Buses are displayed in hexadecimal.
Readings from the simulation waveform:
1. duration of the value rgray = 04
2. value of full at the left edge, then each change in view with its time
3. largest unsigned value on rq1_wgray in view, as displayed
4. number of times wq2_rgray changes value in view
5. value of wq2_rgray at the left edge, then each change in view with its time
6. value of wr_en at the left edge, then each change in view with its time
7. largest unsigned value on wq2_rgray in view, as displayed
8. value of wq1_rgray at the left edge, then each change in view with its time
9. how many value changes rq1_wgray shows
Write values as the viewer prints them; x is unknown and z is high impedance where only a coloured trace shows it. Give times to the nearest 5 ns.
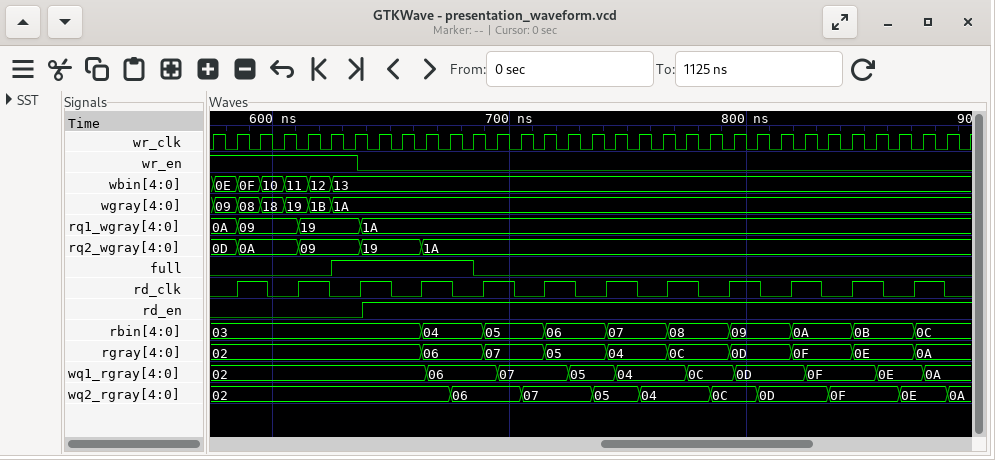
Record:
25 ns
0, 1 at 625 ns, 0 at 685 ns
1A
9
02, 06 at 675 ns, 07 at 705 ns, 05 at 735 ns, 04 at 755 ns, 0C at 785 ns, 0D at 805 ns, 0F at 835 ns, 0E at 865 ns, 0A at 885 ns
1, 0 at 635 ns
0F
02, 06 at 665 ns, 07 at 695 ns, 05 at 725 ns, 04 at 745 ns, 0C at 775 ns, 0D at 795 ns, 0F at 825 ns, 0E at 855 ns, 0A at 875 ns
3
